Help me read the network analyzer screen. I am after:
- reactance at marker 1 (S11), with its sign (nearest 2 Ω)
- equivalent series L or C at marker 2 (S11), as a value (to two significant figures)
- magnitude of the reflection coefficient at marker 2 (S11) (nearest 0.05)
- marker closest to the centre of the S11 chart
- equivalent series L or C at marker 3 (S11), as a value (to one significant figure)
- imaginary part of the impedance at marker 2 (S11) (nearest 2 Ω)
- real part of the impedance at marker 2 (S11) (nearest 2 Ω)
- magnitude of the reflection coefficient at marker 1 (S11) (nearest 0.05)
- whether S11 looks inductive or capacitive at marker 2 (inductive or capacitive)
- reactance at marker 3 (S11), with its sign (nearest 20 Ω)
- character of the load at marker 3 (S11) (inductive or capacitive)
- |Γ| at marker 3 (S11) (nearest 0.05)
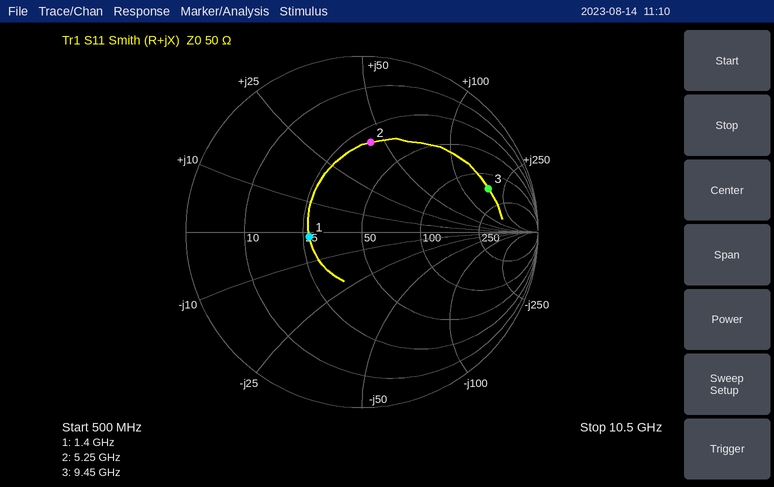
-2 Ω
1.3 nH
0.50
marker 1
3 nH
+44 Ω
32 Ω
0.30
inductive
+180 Ω
inductive
0.75
